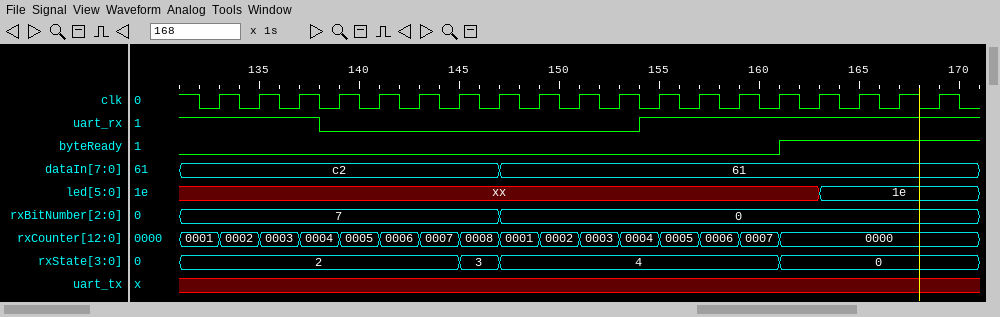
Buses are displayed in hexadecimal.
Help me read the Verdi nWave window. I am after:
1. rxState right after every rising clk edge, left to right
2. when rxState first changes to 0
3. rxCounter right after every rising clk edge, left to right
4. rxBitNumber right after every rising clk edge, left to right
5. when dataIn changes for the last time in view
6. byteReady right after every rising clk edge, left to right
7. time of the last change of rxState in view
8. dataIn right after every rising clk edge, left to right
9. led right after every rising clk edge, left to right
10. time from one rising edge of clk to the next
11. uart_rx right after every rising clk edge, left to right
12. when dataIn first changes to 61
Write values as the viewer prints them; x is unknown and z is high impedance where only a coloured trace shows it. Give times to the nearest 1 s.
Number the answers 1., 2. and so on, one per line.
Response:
1. 2, 2, 2, 2, 2, 2, 3, 4, 4, 4, 4, 4, 4, 4, 0, 0, 0, 0, 0
2. 161 s
3. 0002, 0003, 0004, 0005, 0006, 0007, 0008, 0001, 0002, 0003, 0004, 0005, 0006, 0007, 0000, 0000, 0000, 0000, 0000
4. 7, 7, 7, 7, 7, 7, 7, 0, 0, 0, 0, 0, 0, 0, 0, 0, 0, 0, 0
5. 147 s
6. 0 0 0 0 0 0 0 0 0 0 0 0 0 0 1 1 1 1 1
7. 161 s
8. c2, c2, c2, c2, c2, c2, c2, 61, 61, 61, 61, 61, 61, 61, 61, 61, 61, 61, 61
9. xx, xx, xx, xx, xx, xx, xx, xx, xx, xx, xx, xx, xx, xx, xx, 1e, 1e, 1e, 1e
10. 2 s
11. 1 1 1 0 0 0 0 0 0 0 0 1 1 1 1 1 1 1 1
12. 147 s
